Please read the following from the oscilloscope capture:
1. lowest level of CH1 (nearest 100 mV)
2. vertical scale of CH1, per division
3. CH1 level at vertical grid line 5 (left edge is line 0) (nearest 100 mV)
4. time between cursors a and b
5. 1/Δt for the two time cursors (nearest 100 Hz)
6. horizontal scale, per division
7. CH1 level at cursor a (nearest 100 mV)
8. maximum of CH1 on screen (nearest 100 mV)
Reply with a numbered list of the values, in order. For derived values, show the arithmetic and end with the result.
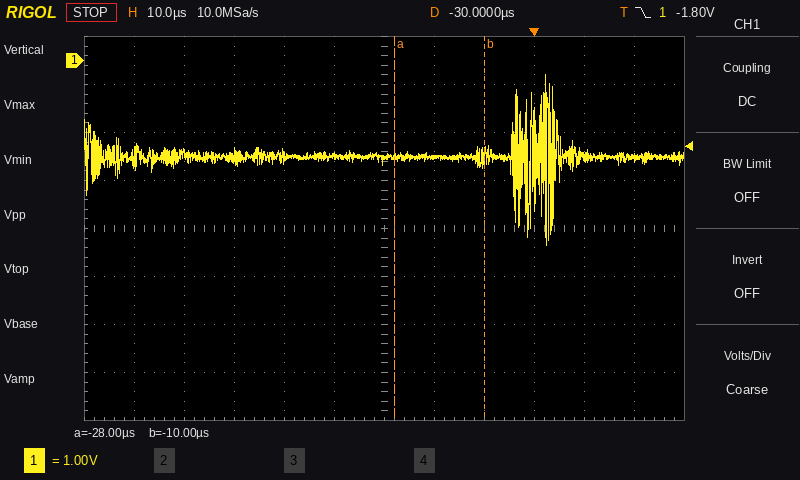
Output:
1. -3.8 V
2. 1 V
3. -2.0 V
4. -10 µs − (-28 µs) = 18 µs
5. 1 / 18 µs ≈ 55.6 kHz
6. 10 µs
7. -2.0 V
8. -300 mV
